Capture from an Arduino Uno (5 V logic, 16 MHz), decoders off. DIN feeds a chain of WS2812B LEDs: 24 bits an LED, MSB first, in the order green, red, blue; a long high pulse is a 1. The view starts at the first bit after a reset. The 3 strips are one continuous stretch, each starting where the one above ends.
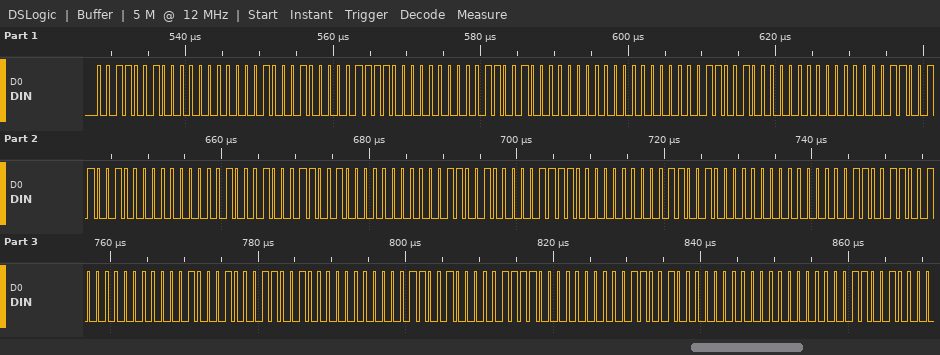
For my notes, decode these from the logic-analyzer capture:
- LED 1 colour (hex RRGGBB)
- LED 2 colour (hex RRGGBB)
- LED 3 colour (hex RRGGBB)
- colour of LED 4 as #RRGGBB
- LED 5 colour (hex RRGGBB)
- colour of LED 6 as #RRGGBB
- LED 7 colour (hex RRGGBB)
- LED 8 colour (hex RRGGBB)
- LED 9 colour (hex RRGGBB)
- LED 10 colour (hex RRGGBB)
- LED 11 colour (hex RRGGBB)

#003222
#000F32
#000032
#030032
#220032
#32000F
#320000
#320300
#322200
#0F3200
#003200
